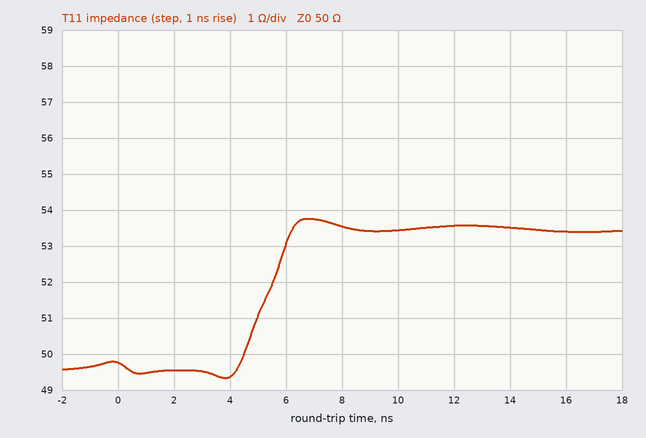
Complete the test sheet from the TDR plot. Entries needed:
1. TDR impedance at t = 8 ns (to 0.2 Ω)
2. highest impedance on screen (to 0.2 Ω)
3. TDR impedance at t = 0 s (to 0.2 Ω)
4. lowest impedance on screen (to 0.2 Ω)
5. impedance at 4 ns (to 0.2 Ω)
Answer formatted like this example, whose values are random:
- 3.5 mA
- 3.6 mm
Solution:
- 53.6 Ω
- 53.8 Ω
- 49.8 Ω
- 49.4 Ω
- 49.4 Ω
